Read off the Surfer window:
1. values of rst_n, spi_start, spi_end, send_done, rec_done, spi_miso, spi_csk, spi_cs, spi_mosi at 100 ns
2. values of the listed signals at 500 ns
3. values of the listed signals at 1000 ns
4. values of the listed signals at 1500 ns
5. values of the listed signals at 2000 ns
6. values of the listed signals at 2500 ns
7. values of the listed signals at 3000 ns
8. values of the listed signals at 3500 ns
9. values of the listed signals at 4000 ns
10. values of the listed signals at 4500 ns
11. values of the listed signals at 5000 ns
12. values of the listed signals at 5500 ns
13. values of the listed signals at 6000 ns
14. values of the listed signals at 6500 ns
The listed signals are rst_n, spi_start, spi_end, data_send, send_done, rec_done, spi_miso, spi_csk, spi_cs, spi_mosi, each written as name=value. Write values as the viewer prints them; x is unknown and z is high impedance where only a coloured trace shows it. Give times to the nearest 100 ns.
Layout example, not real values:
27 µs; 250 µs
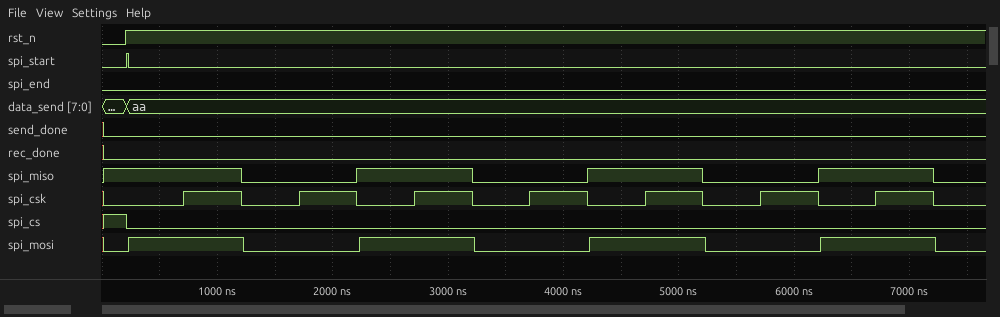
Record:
rst_n=0, spi_start=0, spi_end=0, send_done=0, rec_done=0, spi_miso=1, spi_csk=0, spi_cs=1, spi_mosi=0; rst_n=1, spi_start=0, spi_end=0, data_send=aa, send_done=0, rec_done=0, spi_miso=1, spi_csk=0, spi_cs=0, spi_mosi=1; rst_n=1, spi_start=0, spi_end=0, data_send=aa, send_done=0, rec_done=0, spi_miso=1, spi_csk=1, spi_cs=0, spi_mosi=1; rst_n=1, spi_start=0, spi_end=0, data_send=aa, send_done=0, rec_done=0, spi_miso=0, spi_csk=0, spi_cs=0, spi_mosi=0; rst_n=1, spi_start=0, spi_end=0, data_send=aa, send_done=0, rec_done=0, spi_miso=0, spi_csk=1, spi_cs=0, spi_mosi=0; rst_n=1, spi_start=0, spi_end=0, data_send=aa, send_done=0, rec_done=0, spi_miso=1, spi_csk=0, spi_cs=0, spi_mosi=1; rst_n=1, spi_start=0, spi_end=0, data_send=aa, send_done=0, rec_done=0, spi_miso=1, spi_csk=1, spi_cs=0, spi_mosi=1; rst_n=1, spi_start=0, spi_end=0, data_send=aa, send_done=0, rec_done=0, spi_miso=0, spi_csk=0, spi_cs=0, spi_mosi=0; rst_n=1, spi_start=0, spi_end=0, data_send=aa, send_done=0, rec_done=0, spi_miso=0, spi_csk=1, spi_cs=0, spi_mosi=0; rst_n=1, spi_start=0, spi_end=0, data_send=aa, send_done=0, rec_done=0, spi_miso=1, spi_csk=0, spi_cs=0, spi_mosi=1; rst_n=1, spi_start=0, spi_end=0, data_send=aa, send_done=0, rec_done=0, spi_miso=1, spi_csk=1, spi_cs=0, spi_mosi=1; rst_n=1, spi_start=0, spi_end=0, data_send=aa, send_done=0, rec_done=0, spi_miso=0, spi_csk=0, spi_cs=0, spi_mosi=0; rst_n=1, spi_start=0, spi_end=0, data_send=aa, send_done=0, rec_done=0, spi_miso=0, spi_csk=1, spi_cs=0, spi_mosi=0; rst_n=1, spi_start=0, spi_end=0, data_send=aa, send_done=0, rec_done=0, spi_miso=1, spi_csk=0, spi_cs=0, spi_mosi=1
